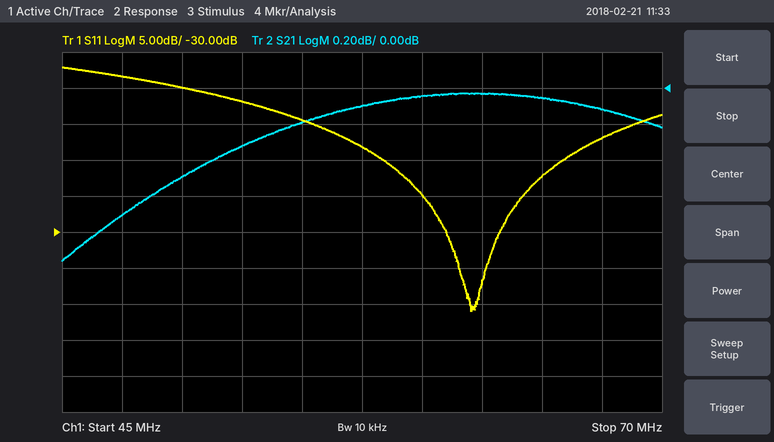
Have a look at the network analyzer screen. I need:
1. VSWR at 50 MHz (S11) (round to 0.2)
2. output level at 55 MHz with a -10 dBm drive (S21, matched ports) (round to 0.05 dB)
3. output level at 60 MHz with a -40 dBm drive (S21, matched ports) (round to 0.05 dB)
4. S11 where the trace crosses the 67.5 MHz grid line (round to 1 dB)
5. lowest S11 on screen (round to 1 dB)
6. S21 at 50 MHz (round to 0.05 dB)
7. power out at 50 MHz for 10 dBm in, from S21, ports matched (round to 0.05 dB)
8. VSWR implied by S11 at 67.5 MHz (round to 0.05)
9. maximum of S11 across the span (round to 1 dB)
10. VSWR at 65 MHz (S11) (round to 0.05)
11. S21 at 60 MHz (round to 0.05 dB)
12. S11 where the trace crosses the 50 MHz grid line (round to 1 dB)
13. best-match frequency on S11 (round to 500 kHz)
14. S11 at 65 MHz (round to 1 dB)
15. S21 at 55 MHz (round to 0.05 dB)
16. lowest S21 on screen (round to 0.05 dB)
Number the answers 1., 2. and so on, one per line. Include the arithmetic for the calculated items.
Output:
1. |Γ| = 10^(-10/20) = 0.3162; VSWR = (1 + 0.3162)/(1 − 0.3162) ≈ 1.92, so 2.0 to the nearest 0.2
2. -10 dBm + (-0.20 dB) = -10.20 dBm
3. -40 dBm + (-0.05 dB) = -40.05 dBm
4. -17 dB
5. -41 dB
6. -0.50 dB
7. 10 dBm + (-0.50 dB) = 9.50 dBm
8. |Γ| = 10^(-17/20) = 0.1413; VSWR = (1 + 0.1413)/(1 − 0.1413) ≈ 1.33, so 1.35 to the nearest 0.05
9. -7 dB
10. |Γ| = 10^(-22/20) = 0.0794; VSWR = (1 + 0.0794)/(1 − 0.0794) ≈ 1.17, so 1.15 to the nearest 0.05
11. -0.05 dB
12. -10 dB
13. 62.0 MHz
14. -22 dB
15. -0.20 dB
16. -0.95 dB
